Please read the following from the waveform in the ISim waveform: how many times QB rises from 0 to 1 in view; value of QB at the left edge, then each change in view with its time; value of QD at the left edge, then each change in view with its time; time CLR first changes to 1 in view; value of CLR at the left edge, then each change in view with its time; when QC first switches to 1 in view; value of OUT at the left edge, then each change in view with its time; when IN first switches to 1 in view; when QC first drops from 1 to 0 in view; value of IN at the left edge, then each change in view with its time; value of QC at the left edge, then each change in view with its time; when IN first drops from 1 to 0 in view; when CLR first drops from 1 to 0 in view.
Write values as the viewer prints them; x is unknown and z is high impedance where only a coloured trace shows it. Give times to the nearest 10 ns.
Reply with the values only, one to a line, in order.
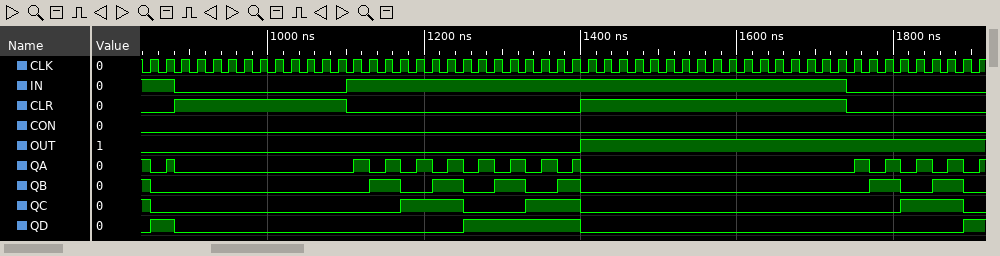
6
1, 0 at 850 ns, 1 at 1130 ns, 0 at 1170 ns, 1 at 1210 ns, 0 at 1250 ns, 1 at 1290 ns, 0 at 1330 ns, 1 at 1370 ns, 0 at 1400 ns, 1 at 1770 ns, 0 at 1810 ns, 1 at 1850 ns, 0 at 1890 ns
0, 1 at 850 ns, 0 at 880 ns, 1 at 1250 ns, 0 at 1400 ns, 1 at 1890 ns
880 ns
0, 1 at 880 ns, 0 at 1100 ns, 1 at 1400 ns, 0 at 1740 ns
1170 ns
0, 1 at 1400 ns
1100 ns
850 ns
1, 0 at 880 ns, 1 at 1100 ns, 0 at 1740 ns
1, 0 at 850 ns, 1 at 1170 ns, 0 at 1250 ns, 1 at 1330 ns, 0 at 1400 ns, 1 at 1810 ns, 0 at 1890 ns
880 ns
1100 ns
